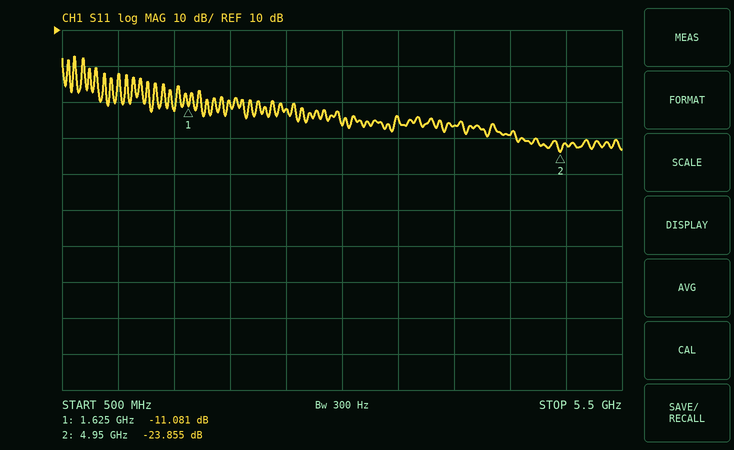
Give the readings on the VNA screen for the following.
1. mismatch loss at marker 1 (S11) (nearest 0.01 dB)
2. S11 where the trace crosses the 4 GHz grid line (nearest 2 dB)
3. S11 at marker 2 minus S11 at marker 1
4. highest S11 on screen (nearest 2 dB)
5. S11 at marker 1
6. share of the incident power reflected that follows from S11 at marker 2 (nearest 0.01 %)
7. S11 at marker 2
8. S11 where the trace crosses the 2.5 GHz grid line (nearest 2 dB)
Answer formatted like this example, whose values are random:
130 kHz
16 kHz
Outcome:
0.35 dB
-16 dB
-12.774 dB
2 dB
-11.081 dB
0.41 %
-23.855 dB
-12 dB
